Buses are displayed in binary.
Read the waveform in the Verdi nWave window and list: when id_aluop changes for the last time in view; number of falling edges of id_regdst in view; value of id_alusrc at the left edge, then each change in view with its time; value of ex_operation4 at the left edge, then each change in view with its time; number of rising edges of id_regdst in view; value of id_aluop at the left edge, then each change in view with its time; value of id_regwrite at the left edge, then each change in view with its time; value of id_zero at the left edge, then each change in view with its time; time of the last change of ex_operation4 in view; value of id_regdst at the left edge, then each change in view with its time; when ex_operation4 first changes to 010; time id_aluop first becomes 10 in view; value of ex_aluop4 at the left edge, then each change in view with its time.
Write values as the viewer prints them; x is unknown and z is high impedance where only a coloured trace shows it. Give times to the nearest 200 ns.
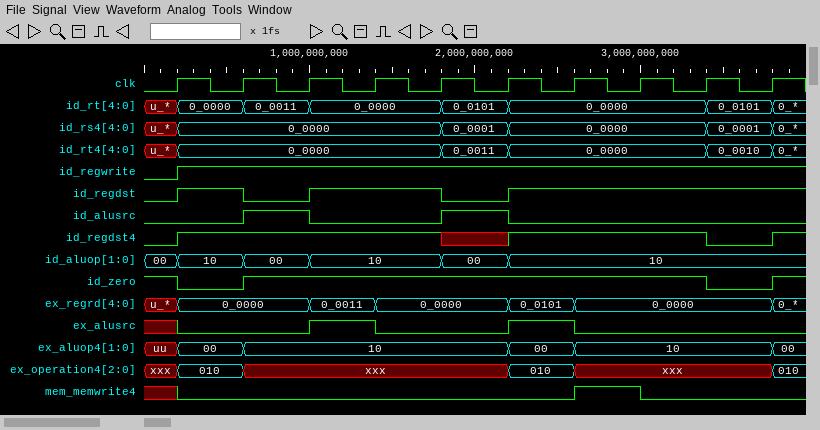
2200 ns
2
0, 1 at 600 ns, 0 at 1000 ns, 1 at 1800 ns, 0 at 2200 ns
xxx, 010 at 200 ns, xxx at 600 ns, 010 at 2200 ns, xxx at 2600 ns, 010 at 3800 ns
3
00, 10 at 200 ns, 00 at 600 ns, 10 at 1000 ns, 00 at 1800 ns, 10 at 2200 ns
0, 1 at 200 ns
1, 0 at 200 ns, 1 at 600 ns, 0 at 3400 ns, 1 at 3800 ns
3800 ns
0, 1 at 200 ns, 0 at 600 ns, 1 at 1000 ns, 0 at 1800 ns, 1 at 2200 ns
200 ns
200 ns
uu, 00 at 200 ns, 10 at 600 ns, 00 at 2200 ns, 10 at 2600 ns, 00 at 3800 ns
